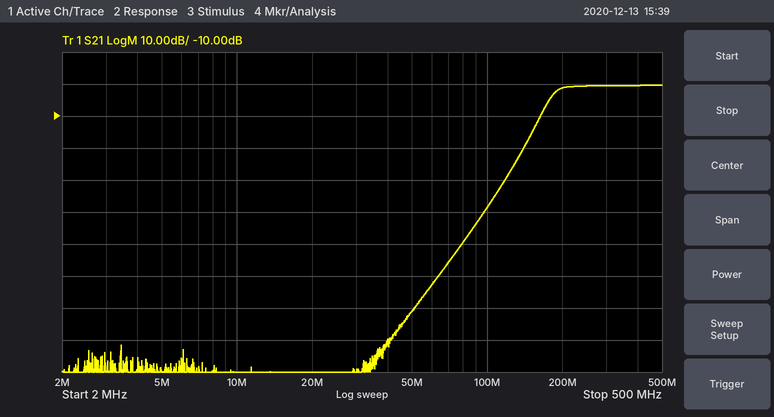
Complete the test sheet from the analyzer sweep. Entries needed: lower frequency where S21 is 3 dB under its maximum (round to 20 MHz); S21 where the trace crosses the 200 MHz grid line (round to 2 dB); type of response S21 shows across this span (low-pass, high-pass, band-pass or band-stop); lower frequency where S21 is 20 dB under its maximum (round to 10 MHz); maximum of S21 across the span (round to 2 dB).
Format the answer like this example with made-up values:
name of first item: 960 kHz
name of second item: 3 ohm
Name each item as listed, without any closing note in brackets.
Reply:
lower frequency where S21 is 3 dB under its maximum: 180 MHz
S21 where the trace crosses the 200 MHz grid line: -2 dB
type of response S21 shows across this span: high-pass
lower frequency where S21 is 20 dB under its maximum: 140 MHz
maximum of S21 across the span: 0 dB
